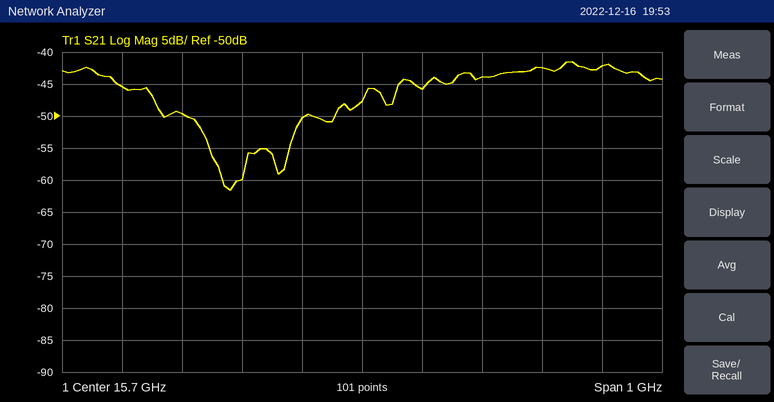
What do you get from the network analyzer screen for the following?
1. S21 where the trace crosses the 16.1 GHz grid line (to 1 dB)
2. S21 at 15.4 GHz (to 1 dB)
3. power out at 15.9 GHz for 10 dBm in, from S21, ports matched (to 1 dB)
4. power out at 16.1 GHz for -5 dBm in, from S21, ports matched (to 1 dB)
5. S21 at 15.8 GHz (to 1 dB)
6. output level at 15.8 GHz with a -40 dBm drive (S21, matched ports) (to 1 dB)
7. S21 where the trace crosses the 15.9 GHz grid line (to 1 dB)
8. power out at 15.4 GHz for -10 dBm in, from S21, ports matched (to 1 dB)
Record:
-42 dB
-50 dB
-34 dBm
-47 dBm
-46 dB
-86 dBm
-44 dB
-60 dBm
